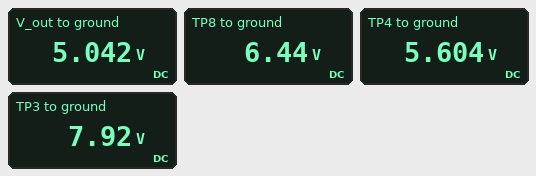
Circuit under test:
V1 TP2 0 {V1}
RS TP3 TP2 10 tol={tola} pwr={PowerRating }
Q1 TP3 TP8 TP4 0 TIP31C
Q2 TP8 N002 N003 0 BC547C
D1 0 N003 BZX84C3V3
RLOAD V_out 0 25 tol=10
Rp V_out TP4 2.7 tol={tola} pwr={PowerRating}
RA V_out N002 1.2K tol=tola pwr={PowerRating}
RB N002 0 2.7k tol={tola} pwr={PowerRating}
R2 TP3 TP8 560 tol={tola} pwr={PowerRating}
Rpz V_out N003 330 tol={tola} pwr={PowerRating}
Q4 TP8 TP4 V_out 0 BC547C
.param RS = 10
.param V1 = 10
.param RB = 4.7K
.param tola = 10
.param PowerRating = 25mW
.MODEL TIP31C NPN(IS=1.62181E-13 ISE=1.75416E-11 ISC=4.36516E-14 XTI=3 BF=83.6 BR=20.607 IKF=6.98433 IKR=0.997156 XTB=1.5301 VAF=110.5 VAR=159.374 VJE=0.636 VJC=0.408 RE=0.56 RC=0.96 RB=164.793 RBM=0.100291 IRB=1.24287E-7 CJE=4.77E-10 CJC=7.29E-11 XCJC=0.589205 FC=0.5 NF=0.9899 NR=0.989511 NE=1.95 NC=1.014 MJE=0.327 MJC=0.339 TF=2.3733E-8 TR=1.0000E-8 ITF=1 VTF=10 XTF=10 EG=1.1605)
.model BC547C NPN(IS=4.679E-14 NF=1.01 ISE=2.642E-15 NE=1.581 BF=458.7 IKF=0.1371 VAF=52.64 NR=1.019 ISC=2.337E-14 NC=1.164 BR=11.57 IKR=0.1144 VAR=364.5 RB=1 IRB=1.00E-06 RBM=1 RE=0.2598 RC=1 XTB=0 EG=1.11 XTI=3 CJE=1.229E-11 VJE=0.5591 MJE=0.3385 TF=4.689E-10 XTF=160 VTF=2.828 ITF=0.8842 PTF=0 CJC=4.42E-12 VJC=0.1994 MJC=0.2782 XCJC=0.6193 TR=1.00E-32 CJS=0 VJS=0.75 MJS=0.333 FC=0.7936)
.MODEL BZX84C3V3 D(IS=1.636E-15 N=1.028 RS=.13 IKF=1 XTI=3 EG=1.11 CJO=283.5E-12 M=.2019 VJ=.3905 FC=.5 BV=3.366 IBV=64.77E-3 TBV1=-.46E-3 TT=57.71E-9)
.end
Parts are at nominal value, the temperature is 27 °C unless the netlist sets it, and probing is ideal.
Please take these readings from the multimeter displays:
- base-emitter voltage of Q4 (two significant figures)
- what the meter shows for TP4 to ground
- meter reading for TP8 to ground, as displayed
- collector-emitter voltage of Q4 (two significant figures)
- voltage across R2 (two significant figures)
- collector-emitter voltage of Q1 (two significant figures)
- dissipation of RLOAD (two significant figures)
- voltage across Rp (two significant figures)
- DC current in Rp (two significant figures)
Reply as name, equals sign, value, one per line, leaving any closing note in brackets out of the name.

base-emitter voltage of Q4 = 560 mV
what the meter shows for TP4 to ground = 5.604 V
meter reading for TP8 to ground, as displayed = 6.44 V
collector-emitter voltage of Q4 = 1.4 V
voltage across R2 = 1.5 V
collector-emitter voltage of Q1 = 2.3 V
dissipation of RLOAD = 1.0 W
voltage across Rp = 560 mV
DC current in Rp = 210 mA
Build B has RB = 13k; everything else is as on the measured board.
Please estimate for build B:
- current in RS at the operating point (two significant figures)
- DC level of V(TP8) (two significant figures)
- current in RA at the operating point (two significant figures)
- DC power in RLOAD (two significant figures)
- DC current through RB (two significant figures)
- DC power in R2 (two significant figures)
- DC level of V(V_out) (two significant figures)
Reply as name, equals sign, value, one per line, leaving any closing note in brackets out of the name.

current in RS at the operating point = 180 mA
DC level of V(TP8) = 5.6 V
current in RA at the operating point = 310 µA
DC power in RLOAD = 750 mW
DC current through RB = 300 µA
DC power in R2 = 12 mW
DC level of V(V_out) = 4.3 V
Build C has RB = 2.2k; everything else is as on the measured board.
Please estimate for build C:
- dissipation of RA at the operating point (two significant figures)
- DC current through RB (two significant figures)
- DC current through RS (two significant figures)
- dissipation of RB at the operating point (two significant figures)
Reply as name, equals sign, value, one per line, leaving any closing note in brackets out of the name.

dissipation of RA at the operating point = 2.6 mW
DC current through RB = 1.5 mA
DC current through RS = 210 mA
dissipation of RB at the operating point = 4.8 mW
